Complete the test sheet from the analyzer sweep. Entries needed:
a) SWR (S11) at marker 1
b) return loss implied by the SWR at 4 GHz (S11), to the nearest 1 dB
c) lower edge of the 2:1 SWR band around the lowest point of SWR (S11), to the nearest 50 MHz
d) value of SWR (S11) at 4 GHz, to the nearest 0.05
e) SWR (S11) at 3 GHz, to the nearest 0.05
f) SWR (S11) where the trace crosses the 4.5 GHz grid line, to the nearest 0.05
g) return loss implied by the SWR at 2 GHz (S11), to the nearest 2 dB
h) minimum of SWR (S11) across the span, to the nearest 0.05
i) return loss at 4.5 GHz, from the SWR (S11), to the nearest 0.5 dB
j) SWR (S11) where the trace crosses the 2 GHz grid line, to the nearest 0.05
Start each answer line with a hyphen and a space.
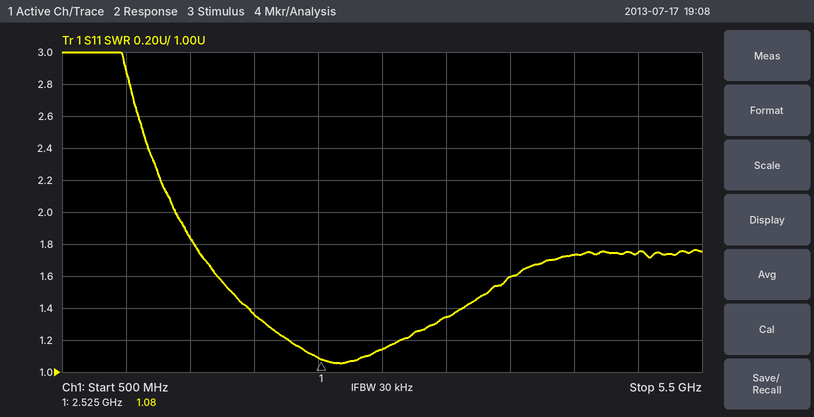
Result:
- 1.08
- 13 dB
- 1.40 GHz
- 1.60
- 1.15
- 1.75
- 16 dB
- 1.05
- 11.5 dB
- 1.35
